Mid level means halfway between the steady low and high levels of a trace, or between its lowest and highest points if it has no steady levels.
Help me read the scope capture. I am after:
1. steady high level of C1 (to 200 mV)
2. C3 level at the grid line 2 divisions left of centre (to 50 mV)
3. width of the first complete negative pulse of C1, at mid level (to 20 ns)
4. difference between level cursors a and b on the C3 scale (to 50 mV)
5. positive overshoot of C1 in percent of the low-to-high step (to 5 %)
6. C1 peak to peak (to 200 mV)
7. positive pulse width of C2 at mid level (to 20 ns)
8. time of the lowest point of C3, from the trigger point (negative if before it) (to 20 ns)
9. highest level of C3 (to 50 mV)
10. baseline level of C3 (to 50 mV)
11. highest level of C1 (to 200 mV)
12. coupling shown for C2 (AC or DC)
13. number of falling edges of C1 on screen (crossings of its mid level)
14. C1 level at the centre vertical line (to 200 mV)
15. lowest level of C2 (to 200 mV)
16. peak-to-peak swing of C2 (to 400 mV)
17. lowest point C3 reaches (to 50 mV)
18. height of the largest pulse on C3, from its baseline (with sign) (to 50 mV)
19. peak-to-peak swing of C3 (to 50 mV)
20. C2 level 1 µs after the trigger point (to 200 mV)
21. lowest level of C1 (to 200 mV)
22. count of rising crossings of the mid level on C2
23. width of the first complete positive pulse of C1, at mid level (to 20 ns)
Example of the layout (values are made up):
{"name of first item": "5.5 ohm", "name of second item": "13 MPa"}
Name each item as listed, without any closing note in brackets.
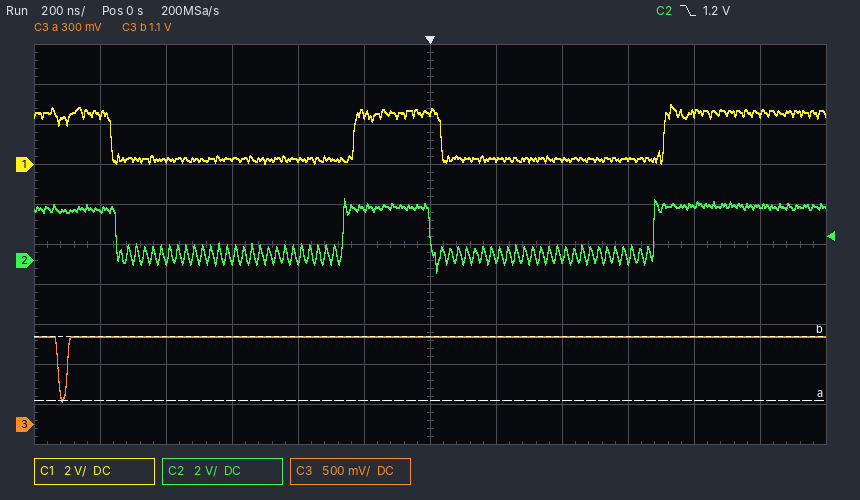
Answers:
{"steady high level of C1": "2.6 V", "C3 level at the grid line 2 divisions left of centre": "1.10 V", "width of the first complete negative pulse of C1, at mid level": "740 ns", "difference between level cursors a and b on the C3 scale": "800 mV", "positive overshoot of C1 in percent of the low-to-high step": "20 %", "C1 peak to peak": "3.0 V", "positive pulse width of C2 at mid level": "260 ns", "time of the lowest point of C3, from the trigger point (negative if before it)": "-1.12 µs", "highest level of C3": "1.10 V", "baseline level of C3": "1.10 V", "highest level of C1": "3.0 V", "coupling shown for C2": "DC", "number of falling edges of C1 on screen": "2", "C1 level at the centre vertical line": "2.6 V", "lowest level of C2": "-600 mV", "peak-to-peak swing of C2": "3.6 V", "lowest point C3 reaches": "300 mV", "height of the largest pulse on C3, from its baseline (with sign)": "-800 mV", "peak-to-peak swing of C3": "800 mV", "C2 level 1 µs after the trigger point": "2.8 V", "lowest level of C1": "0.0 V", "count of rising crossings of the mid level on C2": "2", "width of the first complete positive pulse of C1, at mid level": "260 ns"}
